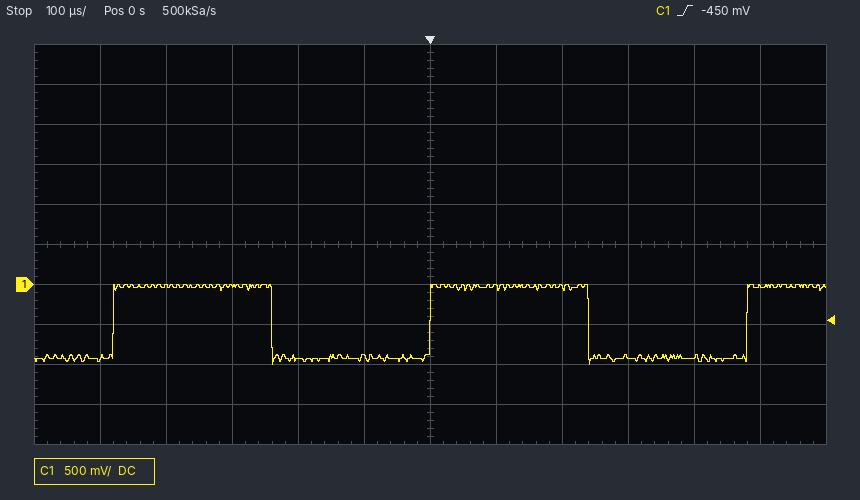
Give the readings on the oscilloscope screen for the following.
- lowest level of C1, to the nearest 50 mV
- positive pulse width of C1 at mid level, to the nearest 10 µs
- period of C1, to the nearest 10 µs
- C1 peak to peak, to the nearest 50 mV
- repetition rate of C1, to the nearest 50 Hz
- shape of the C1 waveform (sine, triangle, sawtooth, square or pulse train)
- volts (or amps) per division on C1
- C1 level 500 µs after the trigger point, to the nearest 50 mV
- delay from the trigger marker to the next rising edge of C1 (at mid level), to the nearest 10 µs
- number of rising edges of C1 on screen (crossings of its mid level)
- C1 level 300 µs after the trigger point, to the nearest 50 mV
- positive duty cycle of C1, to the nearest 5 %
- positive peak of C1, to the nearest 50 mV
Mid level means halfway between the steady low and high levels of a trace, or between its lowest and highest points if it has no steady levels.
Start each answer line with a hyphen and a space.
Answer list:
- -1.00 V
- 240 µs
- 480 µs
- 1.00 V
- 2.10 kHz
- square
- 500 mV
- 0 mV
- 480 µs
- 3
- -900 mV
- 50 %
- 0 mV
